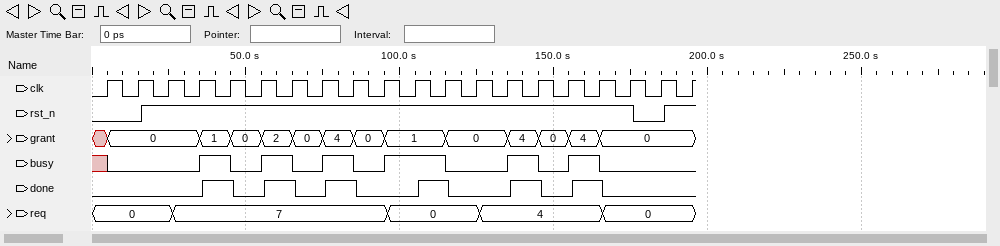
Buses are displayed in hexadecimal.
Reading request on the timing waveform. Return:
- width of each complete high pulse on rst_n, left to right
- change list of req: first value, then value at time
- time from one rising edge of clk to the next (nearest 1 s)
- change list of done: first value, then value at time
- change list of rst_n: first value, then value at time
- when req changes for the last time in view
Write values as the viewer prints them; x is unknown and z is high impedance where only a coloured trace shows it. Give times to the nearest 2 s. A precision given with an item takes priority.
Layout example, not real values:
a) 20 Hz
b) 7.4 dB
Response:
a) 160 s
b) 0, 7 at 26 s, 0 at 96 s, 4 at 126 s, 0 at 166 s
c) 10 s
d) 0, 1 at 36 s, 0 at 46 s, 1 at 56 s, 0 at 66 s, 1 at 76 s, 0 at 86 s, 1 at 106 s, 0 at 116 s, 1 at 136 s, 0 at 146 s, 1 at 156 s, 0 at 166 s
e) 0, 1 at 16 s, 0 at 176 s, 1 at 186 s
f) 166 s
